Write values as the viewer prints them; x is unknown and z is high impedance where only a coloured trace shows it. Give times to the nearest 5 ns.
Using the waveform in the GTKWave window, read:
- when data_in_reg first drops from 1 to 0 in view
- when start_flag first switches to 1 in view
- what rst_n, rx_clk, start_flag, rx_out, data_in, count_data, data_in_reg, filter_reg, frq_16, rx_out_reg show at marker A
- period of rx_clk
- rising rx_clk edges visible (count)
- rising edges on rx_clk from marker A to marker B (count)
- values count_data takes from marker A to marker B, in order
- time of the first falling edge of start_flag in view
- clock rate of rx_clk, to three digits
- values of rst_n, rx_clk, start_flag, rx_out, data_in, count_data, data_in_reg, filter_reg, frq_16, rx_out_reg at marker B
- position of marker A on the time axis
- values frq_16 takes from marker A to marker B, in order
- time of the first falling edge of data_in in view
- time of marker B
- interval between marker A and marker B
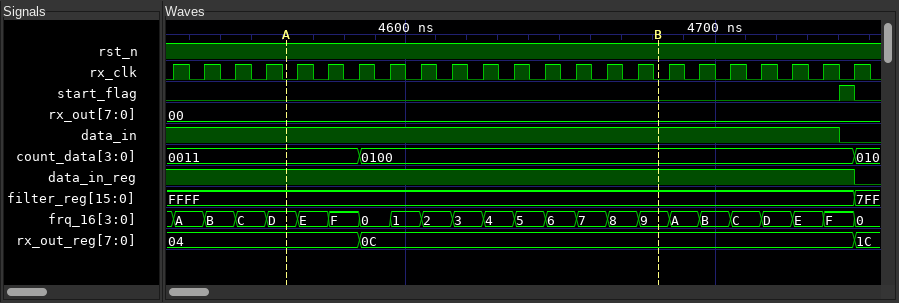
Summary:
4745 ns
4740 ns
rst_n=1, rx_clk=0, start_flag=0, rx_out=00, data_in=1, count_data=0011, data_in_reg=1, filter_reg=FFFF, frq_16=D, rx_out_reg=04
10 ns
23
12
0011, 0100
4745 ns
100 MHz
rst_n=1, rx_clk=0, start_flag=0, rx_out=00, data_in=1, count_data=0100, data_in_reg=1, filter_reg=FFFF, frq_16=9, rx_out_reg=0C
4560 ns
D, E, F, 0, 1, 2, 3, 4, 5, 6, 7, 8, 9
4740 ns
4680 ns
120 ns
